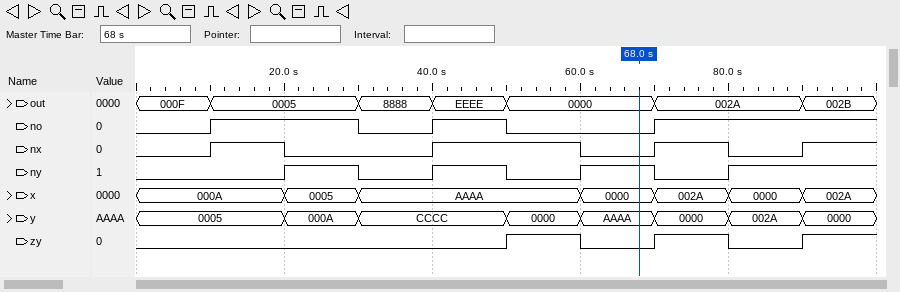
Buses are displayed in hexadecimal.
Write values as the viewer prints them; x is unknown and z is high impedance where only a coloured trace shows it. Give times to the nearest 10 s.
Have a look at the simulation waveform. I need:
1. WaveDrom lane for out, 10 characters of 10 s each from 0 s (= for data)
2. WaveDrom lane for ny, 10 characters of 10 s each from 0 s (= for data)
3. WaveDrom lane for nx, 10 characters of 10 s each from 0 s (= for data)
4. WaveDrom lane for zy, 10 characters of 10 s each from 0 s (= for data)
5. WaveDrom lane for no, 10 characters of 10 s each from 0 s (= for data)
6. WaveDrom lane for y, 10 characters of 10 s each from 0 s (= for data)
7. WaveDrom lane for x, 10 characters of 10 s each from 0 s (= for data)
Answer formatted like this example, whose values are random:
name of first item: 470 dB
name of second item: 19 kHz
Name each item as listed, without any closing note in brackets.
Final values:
WaveDrom lane for out, 10 characters of 10 s each from 0 s: {name: 'out', wave: '==.===.=.=', data: '000F 0005 8888 EEEE 0000 002A 002B'}
WaveDrom lane for ny, 10 characters of 10 s each from 0 s: {name: 'ny', wave: '0.1010101.'}
WaveDrom lane for nx, 10 characters of 10 s each from 0 s: {name: 'nx', wave: '010.1.0101'}
WaveDrom lane for zy, 10 characters of 10 s each from 0 s: {name: 'zy', wave: '0....10101'}
WaveDrom lane for no, 10 characters of 10 s each from 0 s: {name: 'no', wave: '01.010.1..'}
WaveDrom lane for y, 10 characters of 10 s each from 0 s: {name: 'y', wave: '=.==.=====', data: '0005 000A CCCC 0000 AAAA 0000 002A 0000'}
WaveDrom lane for x, 10 characters of 10 s each from 0 s: {name: 'x', wave: '=.==..====', data: '000A 0005 AAAA 0000 002A 0000 002A'}
